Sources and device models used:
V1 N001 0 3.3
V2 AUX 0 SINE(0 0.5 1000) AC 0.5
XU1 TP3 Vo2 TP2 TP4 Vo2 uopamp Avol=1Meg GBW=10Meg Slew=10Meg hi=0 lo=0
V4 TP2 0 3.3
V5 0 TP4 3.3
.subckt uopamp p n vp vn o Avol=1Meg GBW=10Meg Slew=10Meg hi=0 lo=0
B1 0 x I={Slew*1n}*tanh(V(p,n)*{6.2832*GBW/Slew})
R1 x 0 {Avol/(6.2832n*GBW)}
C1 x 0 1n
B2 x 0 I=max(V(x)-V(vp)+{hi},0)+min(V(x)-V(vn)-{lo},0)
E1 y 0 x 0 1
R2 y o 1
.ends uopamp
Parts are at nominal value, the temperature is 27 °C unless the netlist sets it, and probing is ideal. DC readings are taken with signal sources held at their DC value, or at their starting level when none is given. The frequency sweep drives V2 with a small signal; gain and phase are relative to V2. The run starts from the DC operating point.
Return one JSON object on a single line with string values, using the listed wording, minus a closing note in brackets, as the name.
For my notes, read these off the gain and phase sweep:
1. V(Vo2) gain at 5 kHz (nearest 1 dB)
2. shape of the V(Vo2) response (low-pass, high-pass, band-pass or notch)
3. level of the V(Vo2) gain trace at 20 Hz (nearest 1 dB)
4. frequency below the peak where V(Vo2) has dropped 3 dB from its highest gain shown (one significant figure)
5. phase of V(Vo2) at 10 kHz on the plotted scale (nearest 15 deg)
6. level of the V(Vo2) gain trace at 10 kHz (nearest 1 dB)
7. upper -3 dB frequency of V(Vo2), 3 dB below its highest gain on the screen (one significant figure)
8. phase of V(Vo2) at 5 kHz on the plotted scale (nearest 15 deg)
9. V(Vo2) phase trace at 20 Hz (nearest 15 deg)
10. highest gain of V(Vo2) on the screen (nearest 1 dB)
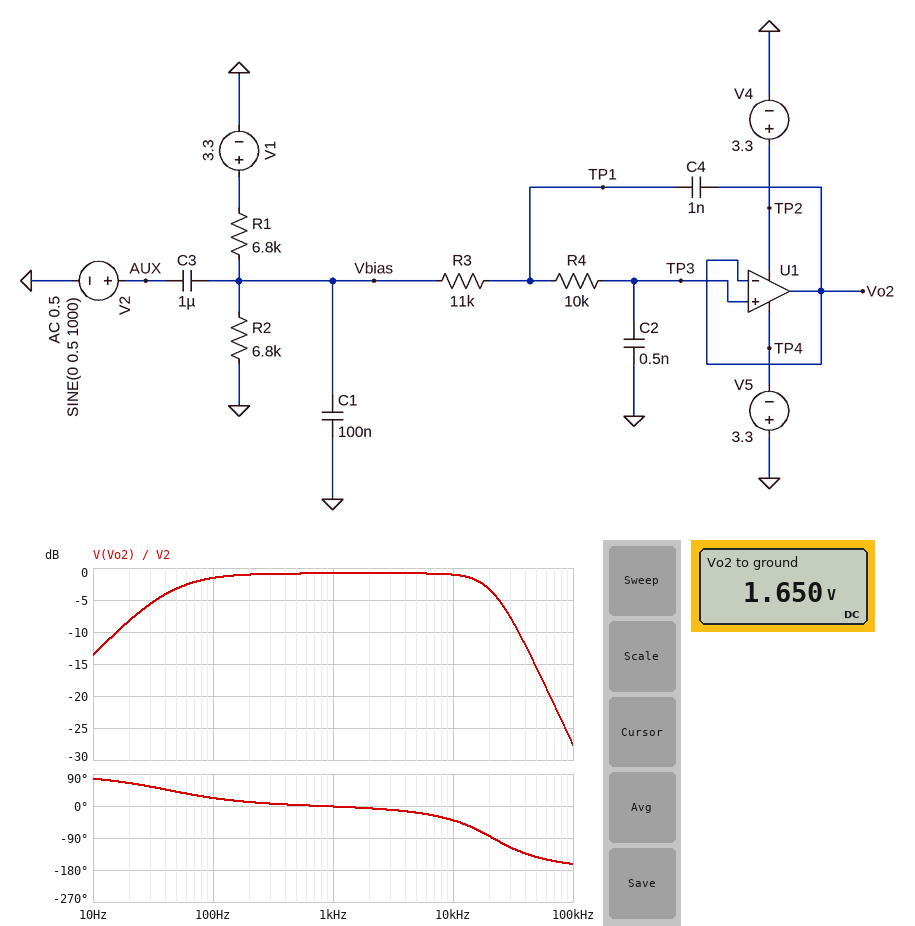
{"V(Vo2) gain at 5 kHz": "-1 dB", "shape of the V(Vo2) response": "band-pass", "level of the V(Vo2) gain trace at 20 Hz": "-8 dB", "frequency below the peak where V(Vo2) has dropped 3 dB from its highest gain shown": "40 Hz", "phase of V(Vo2) at 10 kHz on the plotted scale": "-45 deg", "level of the V(Vo2) gain trace at 10 kHz": "-1 dB", "upper -3 dB frequency of V(Vo2), 3 dB below its highest gain on the screen": "20 kHz", "phase of V(Vo2) at 5 kHz on the plotted scale": "-15 deg", "V(Vo2) phase trace at 20 Hz": "60 deg", "highest gain of V(Vo2) on the screen": "-1 dB"}
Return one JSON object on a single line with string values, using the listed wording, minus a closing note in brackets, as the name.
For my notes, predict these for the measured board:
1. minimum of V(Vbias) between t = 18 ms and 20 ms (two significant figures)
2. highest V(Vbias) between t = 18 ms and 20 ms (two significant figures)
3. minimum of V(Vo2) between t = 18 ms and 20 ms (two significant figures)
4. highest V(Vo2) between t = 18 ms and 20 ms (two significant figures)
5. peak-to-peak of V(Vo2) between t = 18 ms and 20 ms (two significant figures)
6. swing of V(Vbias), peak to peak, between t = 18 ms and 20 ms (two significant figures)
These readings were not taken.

{"minimum of V(Vbias) between t = 18 ms and 20 ms": "1.2 V", "highest V(Vbias) between t = 18 ms and 20 ms": "2.1 V", "minimum of V(Vo2) between t = 18 ms and 20 ms": "1.2 V", "highest V(Vo2) between t = 18 ms and 20 ms": "2.1 V", "peak-to-peak of V(Vo2) between t = 18 ms and 20 ms": "910 mV", "swing of V(Vbias), peak to peak, between t = 18 ms and 20 ms": "910 mV"}
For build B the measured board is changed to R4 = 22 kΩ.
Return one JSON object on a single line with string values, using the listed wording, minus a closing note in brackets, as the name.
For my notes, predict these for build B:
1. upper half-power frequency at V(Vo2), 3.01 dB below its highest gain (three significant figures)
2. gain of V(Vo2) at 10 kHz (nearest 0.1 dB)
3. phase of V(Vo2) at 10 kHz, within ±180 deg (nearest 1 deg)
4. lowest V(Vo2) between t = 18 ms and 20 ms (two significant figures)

{"upper half-power frequency at V(Vo2), 3.01 dB below its highest gain": "13.6 kHz", "gain of V(Vo2) at 10 kHz": "-2.1 dB", "phase of V(Vo2) at 10 kHz, within ±180 deg": "-63 deg", "lowest V(Vo2) between t = 18 ms and 20 ms": "1.2 V"}
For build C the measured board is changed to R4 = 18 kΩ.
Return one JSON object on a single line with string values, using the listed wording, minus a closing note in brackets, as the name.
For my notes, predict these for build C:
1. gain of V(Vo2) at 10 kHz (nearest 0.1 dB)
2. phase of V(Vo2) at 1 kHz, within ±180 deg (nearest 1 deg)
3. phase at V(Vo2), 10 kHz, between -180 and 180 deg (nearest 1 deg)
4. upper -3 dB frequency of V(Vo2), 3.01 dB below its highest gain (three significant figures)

{"gain of V(Vo2) at 10 kHz": "-1.6 dB", "phase of V(Vo2) at 1 kHz, within ±180 deg": "-3 deg", "phase at V(Vo2), 10 kHz, between -180 and 180 deg": "-56 deg", "upper -3 dB frequency of V(Vo2), 3.01 dB below its highest gain": "15.5 kHz"}
